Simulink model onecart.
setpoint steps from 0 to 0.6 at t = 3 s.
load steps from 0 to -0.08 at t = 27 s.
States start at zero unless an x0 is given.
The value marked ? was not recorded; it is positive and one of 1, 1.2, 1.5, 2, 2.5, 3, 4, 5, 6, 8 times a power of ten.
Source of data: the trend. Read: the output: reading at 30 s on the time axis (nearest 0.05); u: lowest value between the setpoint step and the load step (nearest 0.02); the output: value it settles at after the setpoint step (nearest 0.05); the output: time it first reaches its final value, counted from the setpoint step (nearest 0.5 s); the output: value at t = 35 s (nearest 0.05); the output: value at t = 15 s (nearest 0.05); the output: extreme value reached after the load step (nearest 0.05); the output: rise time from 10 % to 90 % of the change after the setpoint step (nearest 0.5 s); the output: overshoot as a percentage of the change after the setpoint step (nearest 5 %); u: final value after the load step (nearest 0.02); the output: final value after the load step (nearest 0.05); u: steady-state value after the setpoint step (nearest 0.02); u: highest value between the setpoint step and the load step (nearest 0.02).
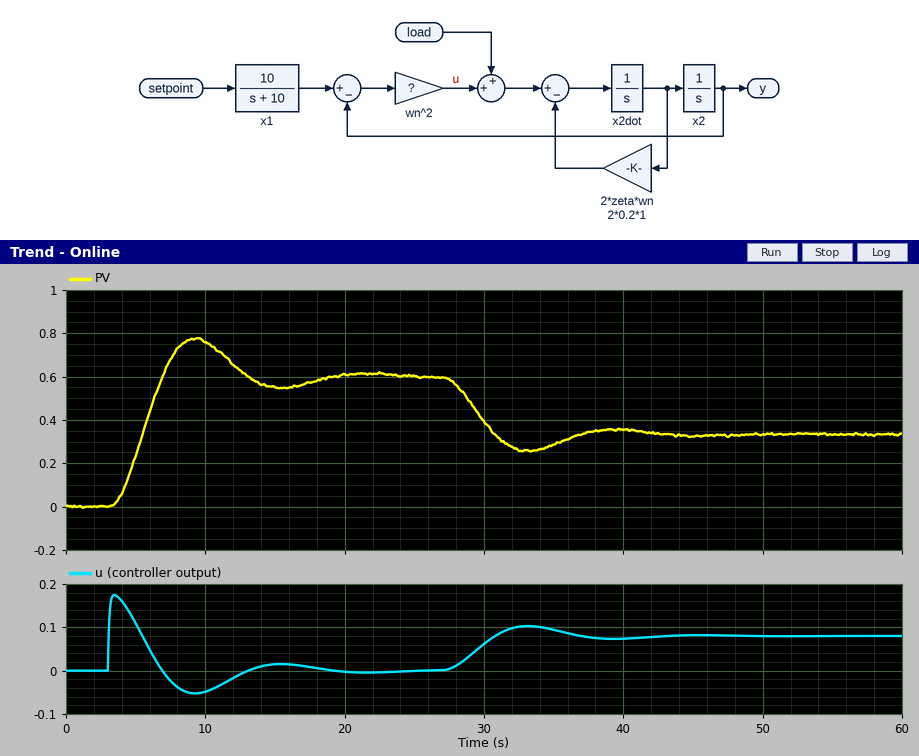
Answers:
0.40
-0.06
0.60
4.0 s
0.30
0.55
0.25
2.5 s
30 %
0.08
0.35
0.00
0.18
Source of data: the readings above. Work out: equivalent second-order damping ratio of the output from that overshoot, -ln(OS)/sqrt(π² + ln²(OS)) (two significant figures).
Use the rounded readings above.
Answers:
0.36
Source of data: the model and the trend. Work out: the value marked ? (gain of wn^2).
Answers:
0.3
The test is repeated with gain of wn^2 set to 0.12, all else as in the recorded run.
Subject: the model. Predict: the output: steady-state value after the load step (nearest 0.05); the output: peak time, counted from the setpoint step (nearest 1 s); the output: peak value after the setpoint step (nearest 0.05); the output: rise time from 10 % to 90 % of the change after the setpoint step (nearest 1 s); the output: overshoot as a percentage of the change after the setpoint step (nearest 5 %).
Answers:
-0.05
11 s
0.65
5 s
10 %
